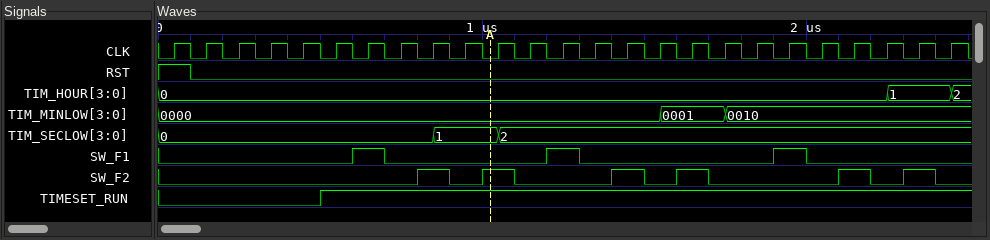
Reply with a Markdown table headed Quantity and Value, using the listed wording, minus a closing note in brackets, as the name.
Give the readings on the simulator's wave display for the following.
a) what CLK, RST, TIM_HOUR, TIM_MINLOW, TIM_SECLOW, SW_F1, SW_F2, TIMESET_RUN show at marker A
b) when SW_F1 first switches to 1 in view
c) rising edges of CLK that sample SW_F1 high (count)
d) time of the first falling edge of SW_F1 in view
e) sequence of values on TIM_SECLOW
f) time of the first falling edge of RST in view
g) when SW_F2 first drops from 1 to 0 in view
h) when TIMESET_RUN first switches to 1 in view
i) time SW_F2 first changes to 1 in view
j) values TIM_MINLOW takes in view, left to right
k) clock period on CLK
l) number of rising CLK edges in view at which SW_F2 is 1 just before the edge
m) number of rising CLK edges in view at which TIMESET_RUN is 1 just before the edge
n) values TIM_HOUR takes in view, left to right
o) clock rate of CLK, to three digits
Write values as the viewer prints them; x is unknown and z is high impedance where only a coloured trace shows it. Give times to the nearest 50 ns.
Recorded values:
| Quantity | Value |
|---|---|
| what CLK, RST, TIM_HOUR, TIM_MINLOW, TIM_SECLOW, SW_F1, SW_F2, TIMESET_RUN show at marker A | CLK=0, RST=0, TIM_HOUR=0, TIM_MINLOW=0000, TIM_SECLOW=1, SW_F1=0, SW_F2=1, TIMESET_RUN=1 |
| when SW_F1 first switches to 1 in view | 600 ns |
| rising edges of CLK that sample SW_F1 high | 3 |
| time of the first falling edge of SW_F1 in view | 700 ns |
| sequence of values on TIM_SECLOW | 0, 1, 2 |
| time of the first falling edge of RST in view | 100 ns |
| when SW_F2 first drops from 1 to 0 in view | 900 ns |
| when TIMESET_RUN first switches to 1 in view | 500 ns |
| time SW_F2 first changes to 1 in view | 800 ns |
| values TIM_MINLOW takes in view, left to right | 0000, 0001, 0010 |
| clock period on CLK | 100 ns |
| number of rising CLK edges in view at which SW_F2 is 1 just before the edge | 6 |
| number of rising CLK edges in view at which TIMESET_RUN is 1 just before the edge | 20 |
| values TIM_HOUR takes in view, left to right | 0, 1, 2 |
| clock rate of CLK, to three digits | 10.0 MHz |
